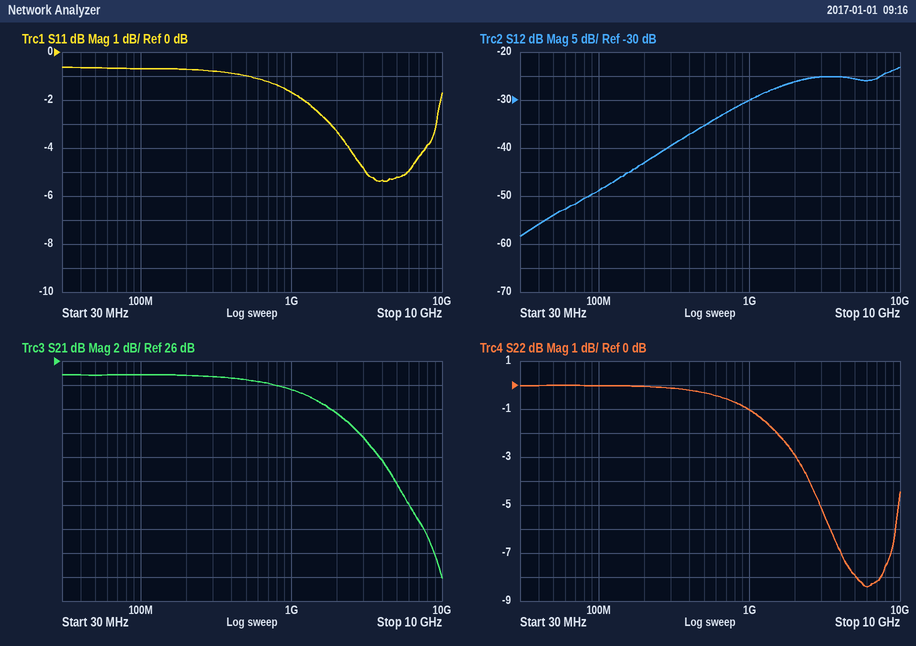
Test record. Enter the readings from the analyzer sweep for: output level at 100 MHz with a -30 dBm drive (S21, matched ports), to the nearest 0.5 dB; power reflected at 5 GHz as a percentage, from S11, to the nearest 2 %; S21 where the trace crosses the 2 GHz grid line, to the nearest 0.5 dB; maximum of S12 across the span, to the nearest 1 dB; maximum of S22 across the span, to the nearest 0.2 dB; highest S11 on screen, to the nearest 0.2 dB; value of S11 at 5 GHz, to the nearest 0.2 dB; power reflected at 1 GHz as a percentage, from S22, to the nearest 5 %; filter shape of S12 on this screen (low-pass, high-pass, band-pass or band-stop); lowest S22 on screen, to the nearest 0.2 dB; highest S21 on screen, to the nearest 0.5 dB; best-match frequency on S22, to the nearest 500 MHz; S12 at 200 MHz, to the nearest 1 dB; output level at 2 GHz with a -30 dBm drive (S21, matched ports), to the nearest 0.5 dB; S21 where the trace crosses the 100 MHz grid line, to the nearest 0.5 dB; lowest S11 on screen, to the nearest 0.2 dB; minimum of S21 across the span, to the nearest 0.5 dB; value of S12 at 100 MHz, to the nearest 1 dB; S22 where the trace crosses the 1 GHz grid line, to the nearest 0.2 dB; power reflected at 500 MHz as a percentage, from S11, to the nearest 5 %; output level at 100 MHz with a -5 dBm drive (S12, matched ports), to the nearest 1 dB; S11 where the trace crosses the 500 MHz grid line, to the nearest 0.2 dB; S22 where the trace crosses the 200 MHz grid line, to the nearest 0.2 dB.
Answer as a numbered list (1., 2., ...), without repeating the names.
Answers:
1. -5.0 dBm
2. 30 %
3. 21.5 dB
4. -23 dB
5. 0.0 dB
6. -0.6 dB
7. -5.2 dB
8. 80 %
9. high-pass
10. -8.4 dB
11. 25.0 dB
12. 6.0 GHz
13. -43 dB
14. -8.5 dBm
15. 25.0 dB
16. -5.4 dB
17. 8.0 dB
18. -49 dB
19. -1.0 dB
20. 80 %
21. -54 dBm
22. -1.0 dB
23. 0.0 dB
